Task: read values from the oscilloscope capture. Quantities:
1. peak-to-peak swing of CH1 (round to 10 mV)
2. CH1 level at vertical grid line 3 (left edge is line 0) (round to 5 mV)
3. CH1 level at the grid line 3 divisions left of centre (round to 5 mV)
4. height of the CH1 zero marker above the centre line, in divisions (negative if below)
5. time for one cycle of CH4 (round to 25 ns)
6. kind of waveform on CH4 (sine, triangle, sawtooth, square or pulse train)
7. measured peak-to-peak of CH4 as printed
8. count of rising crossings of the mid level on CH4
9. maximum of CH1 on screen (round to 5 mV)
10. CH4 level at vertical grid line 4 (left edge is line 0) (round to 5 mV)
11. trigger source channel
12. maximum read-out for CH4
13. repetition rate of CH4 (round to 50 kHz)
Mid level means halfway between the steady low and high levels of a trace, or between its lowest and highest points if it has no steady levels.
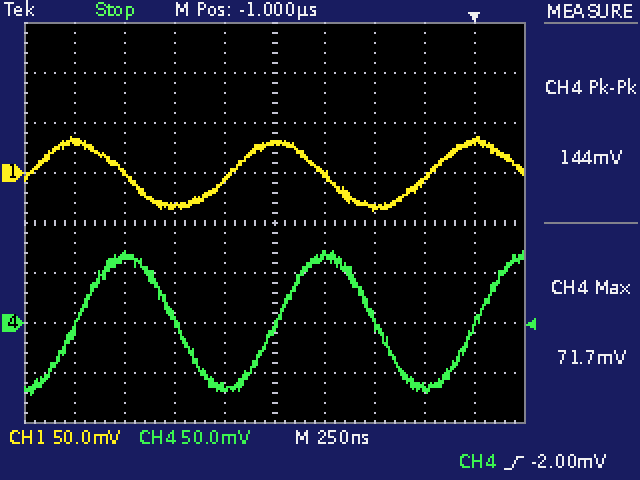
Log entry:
70 mV
-35 mV
0 mV
+1.0 div
1.000 µs
sine
144 mV
3
35 mV
-65 mV
CH4
71.7 mV
1.00 MHz
